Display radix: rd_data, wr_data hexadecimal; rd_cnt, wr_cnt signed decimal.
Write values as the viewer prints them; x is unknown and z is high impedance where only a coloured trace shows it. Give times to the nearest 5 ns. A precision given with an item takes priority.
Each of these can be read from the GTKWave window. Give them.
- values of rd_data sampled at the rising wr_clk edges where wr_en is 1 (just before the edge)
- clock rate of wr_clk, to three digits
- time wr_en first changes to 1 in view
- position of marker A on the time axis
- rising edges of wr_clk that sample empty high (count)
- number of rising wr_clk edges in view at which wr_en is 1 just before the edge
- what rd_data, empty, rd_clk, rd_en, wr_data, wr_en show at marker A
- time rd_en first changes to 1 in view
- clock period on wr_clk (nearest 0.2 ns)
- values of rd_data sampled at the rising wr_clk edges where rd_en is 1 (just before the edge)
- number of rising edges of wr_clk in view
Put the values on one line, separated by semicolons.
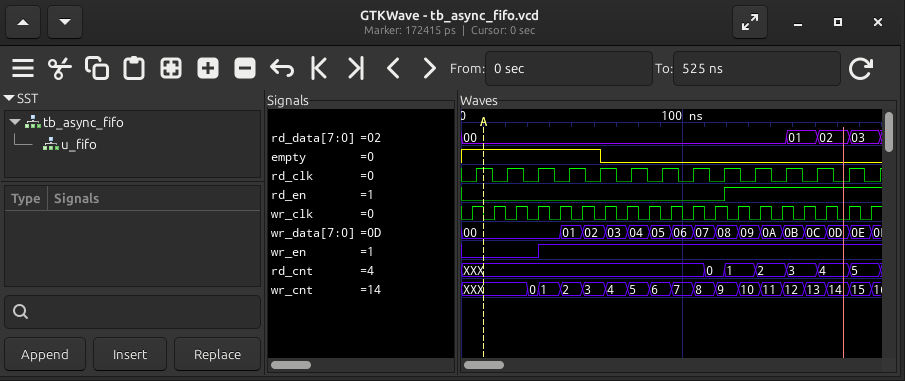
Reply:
00, 00, 00, 00, 00, 00, 00, 00, 00, 00, 00, 01, 02, 02, 03; 100 MHz; 35 ns; 10 ns; 6; 15; rd_data=00, empty=1, rd_clk=1, rd_en=0, wr_data=00, wr_en=0; 120 ns; 10 ns; 00, 00, 00, 01, 02, 02, 03; 19
